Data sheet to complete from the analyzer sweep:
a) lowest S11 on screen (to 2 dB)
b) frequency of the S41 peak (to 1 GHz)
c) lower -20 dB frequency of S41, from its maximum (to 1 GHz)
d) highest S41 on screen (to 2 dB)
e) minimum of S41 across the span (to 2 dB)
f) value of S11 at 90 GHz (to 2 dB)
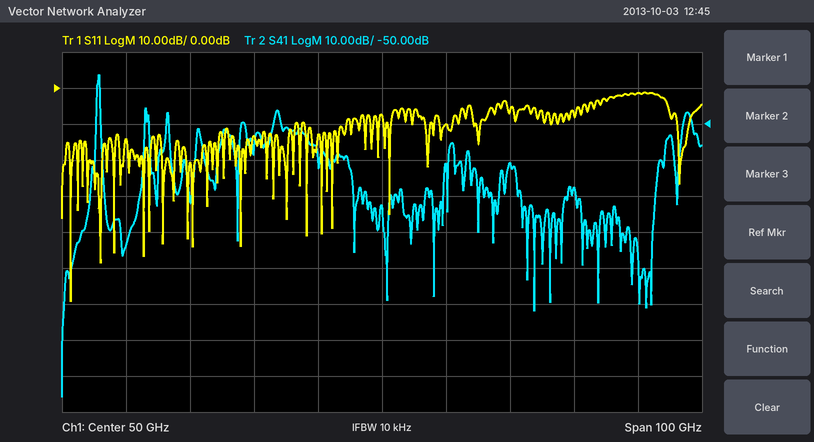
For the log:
-60 dB
6 GHz
5 GHz
-36 dB
-126 dB
-2 dB
